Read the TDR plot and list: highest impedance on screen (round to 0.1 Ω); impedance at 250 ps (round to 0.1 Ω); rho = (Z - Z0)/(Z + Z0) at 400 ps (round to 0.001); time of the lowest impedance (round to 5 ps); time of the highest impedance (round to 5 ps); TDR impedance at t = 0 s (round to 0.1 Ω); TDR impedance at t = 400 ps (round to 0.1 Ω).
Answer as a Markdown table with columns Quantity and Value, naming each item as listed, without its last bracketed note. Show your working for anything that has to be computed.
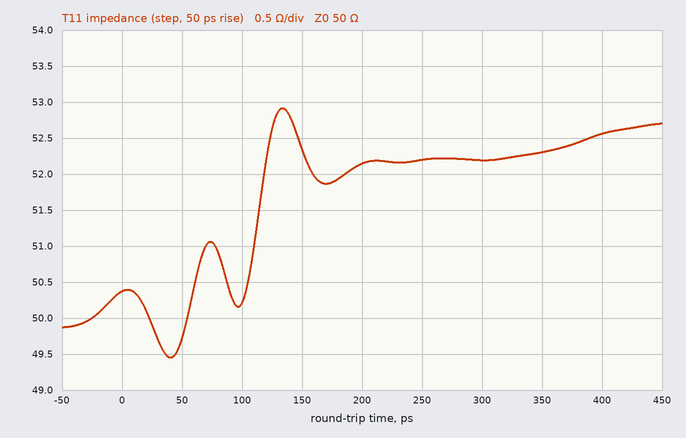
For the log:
| Quantity | Value |
|---|---|
| highest impedance on screen | 52.9 Ω |
| impedance at 250 ps | 52.2 Ω |
| rho = (Z - Z0)/(Z + Z0) at 400 ps | (52.6 − 50)/(52.6 + 50) ≈ +0.025 |
| time of the lowest impedance | 40 ps |
| time of the highest impedance | 135 ps |
| TDR impedance at t = 0 s | 50.4 Ω |
| TDR impedance at t = 400 ps | 52.6 Ω |
